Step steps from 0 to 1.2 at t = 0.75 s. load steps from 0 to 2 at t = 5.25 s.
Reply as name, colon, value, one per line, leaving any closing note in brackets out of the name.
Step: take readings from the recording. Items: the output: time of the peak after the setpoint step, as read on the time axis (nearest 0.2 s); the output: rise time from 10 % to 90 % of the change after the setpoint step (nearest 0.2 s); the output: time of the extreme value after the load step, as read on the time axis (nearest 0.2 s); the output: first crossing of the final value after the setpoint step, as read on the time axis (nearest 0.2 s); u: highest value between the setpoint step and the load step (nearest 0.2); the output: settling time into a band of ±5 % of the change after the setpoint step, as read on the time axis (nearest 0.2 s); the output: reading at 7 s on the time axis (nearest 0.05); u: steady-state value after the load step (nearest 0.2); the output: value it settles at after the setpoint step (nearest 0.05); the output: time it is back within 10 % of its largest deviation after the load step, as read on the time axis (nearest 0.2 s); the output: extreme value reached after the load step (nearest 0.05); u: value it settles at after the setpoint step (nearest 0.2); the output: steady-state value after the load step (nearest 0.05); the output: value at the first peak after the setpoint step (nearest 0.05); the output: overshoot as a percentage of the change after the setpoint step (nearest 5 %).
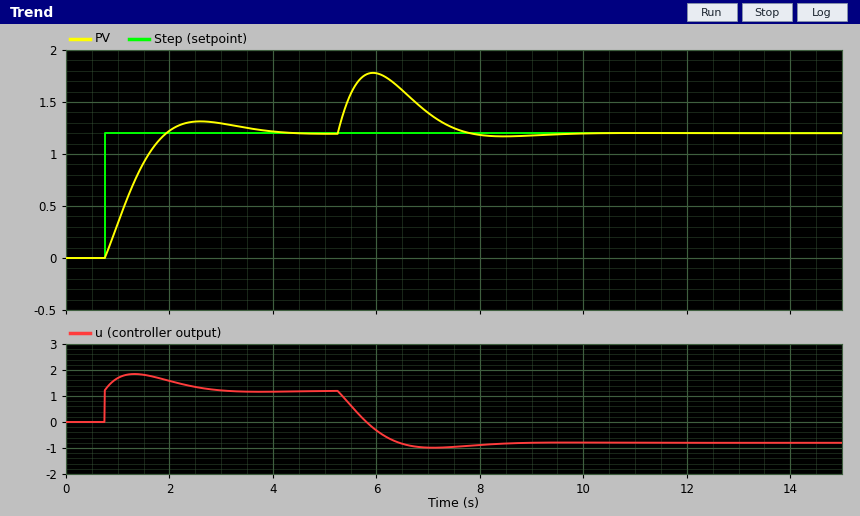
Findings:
the output: time of the peak after the setpoint step, as read on the time axis: 2.6 s
the output: rise time from 10 % to 90 % of the change after the setpoint step: 0.8 s
the output: time of the extreme value after the load step, as read on the time axis: 6.0 s
the output: first crossing of the final value after the setpoint step, as read on the time axis: 2.0 s
u: highest value between the setpoint step and the load step: 1.8
the output: settling time into a band of ±5 % of the change after the setpoint step, as read on the time axis: 3.4 s
the output: reading at 7 s on the time axis: 1.40
u: steady-state value after the load step: -0.8
the output: value it settles at after the setpoint step: 1.20
the output: time it is back within 10 % of its largest deviation after the load step, as read on the time axis: 7.4 s
the output: extreme value reached after the load step: 1.80
u: value it settles at after the setpoint step: 1.2
the output: steady-state value after the load step: 1.20
the output: value at the first peak after the setpoint step: 1.30
the output: overshoot as a percentage of the change after the setpoint step: 10 %
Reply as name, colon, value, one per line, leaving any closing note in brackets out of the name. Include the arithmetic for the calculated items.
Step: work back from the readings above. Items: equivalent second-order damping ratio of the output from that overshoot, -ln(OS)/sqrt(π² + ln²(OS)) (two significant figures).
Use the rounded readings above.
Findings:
equivalent second-order damping ratio of the output from that overshoot, -ln(OS)/sqrt(π² + ln²(OS)): ln(0.1) = -2.303; 2.303 / sqrt(9.870 + 5.302) = 0.59
